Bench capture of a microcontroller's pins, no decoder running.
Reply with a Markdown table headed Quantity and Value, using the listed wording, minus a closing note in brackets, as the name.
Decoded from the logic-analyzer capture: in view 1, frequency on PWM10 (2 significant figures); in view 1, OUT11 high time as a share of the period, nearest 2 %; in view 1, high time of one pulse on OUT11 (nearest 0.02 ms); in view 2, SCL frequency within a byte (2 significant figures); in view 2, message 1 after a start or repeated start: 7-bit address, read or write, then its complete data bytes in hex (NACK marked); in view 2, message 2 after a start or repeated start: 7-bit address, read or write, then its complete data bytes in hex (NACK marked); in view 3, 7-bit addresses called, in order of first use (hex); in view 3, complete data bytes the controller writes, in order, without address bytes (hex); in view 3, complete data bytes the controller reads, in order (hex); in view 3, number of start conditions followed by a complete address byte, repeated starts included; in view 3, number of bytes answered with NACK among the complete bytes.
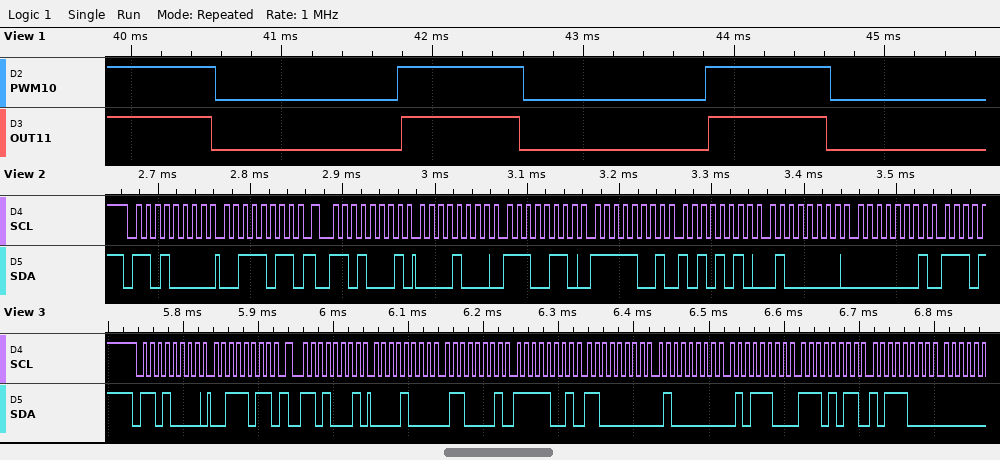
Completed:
| Quantity | Value |
|---|---|
| in view 1, frequency on PWM10 | 490 Hz |
| in view 1, OUT11 high time as a share of the period, nearest 2 % | 38 % |
| in view 1, high time of one pulse on OUT11 | 0.78 ms |
| in view 2, SCL frequency within a byte | 100 kHz |
| in view 2, message 1 after a start or repeated start: 7-bit address, read or write, then its complete data bytes in hex | 0x68 write: 3B |
| in view 2, message 2 after a start or repeated start: 7-bit address, read or write, then its complete data bytes in hex | 0x68 read: 08 E6 F9 AA 40 01 |
| in view 3, 7-bit addresses called, in order of first use | 0x68 |
| in view 3, complete data bytes the controller writes, in order, without address bytes | 3B |
| in view 3, complete data bytes the controller reads, in order | 08 61 F9 C0 40 5C EB B8 |
| in view 3, number of start conditions followed by a complete address byte, repeated starts included | 2 |
| in view 3, number of bytes answered with NACK among the complete bytes | 0 |
